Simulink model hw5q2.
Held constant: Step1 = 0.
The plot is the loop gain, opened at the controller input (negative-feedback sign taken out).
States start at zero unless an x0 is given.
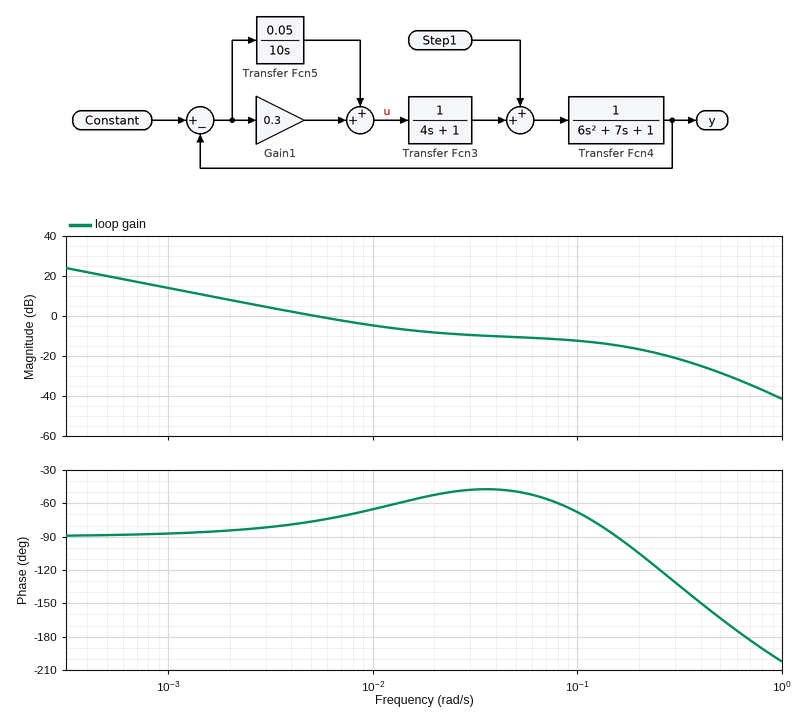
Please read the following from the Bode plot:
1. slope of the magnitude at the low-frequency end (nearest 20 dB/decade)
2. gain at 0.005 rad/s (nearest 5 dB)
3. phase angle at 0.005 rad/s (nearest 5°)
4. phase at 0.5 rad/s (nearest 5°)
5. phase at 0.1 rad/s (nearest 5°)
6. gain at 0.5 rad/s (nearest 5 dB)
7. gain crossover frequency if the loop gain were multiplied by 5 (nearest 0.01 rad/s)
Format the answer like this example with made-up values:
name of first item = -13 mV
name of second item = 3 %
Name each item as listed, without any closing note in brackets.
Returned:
slope of the magnitude at the low-frequency end = -20 dB/decade
gain at 0.005 rad/s = 0 dB
phase angle at 0.005 rad/s = -75°
phase at 0.5 rad/s = -165°
phase at 0.1 rad/s = -70°
gain at 0.5 rad/s = -30 dB
gain crossover frequency if the loop gain were multiplied by 5 = 0.14 rad/s
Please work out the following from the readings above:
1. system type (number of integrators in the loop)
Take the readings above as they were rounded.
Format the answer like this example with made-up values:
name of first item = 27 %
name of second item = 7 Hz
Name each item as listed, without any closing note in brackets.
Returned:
system type = 1
